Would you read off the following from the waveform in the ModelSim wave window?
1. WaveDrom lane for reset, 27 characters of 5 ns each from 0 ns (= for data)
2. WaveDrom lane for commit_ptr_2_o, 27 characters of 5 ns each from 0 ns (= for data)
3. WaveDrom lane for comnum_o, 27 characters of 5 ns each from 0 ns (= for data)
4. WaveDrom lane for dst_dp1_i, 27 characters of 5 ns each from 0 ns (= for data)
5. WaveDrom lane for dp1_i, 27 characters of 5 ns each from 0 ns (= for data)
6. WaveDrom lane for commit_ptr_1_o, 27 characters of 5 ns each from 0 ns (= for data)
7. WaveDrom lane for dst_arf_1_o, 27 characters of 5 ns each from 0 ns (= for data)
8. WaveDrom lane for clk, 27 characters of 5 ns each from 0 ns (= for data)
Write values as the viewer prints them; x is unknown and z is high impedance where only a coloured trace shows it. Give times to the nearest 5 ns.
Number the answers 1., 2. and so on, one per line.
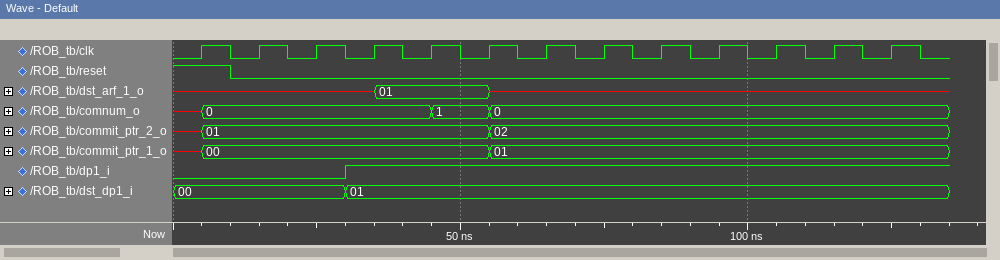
1. {name: 'reset', wave: '1.0........................'}
2. {name: 'commit_ptr_2_o', wave: 'x=.........=...............', data: '01 02'}
3. {name: 'comnum_o', wave: 'x=.......=.=...............', data: '0 1 0'}
4. {name: 'dst_dp1_i', wave: '=.....=....................', data: '00 01'}
5. {name: 'dp1_i', wave: '0.....1....................'}
6. {name: 'commit_ptr_1_o', wave: 'x=.........=...............', data: '00 01'}
7. {name: 'dst_arf_1_o', wave: 'x......=...x...............', data: '01'}
8. {name: 'clk', wave: '010101010101010101010101010'}
